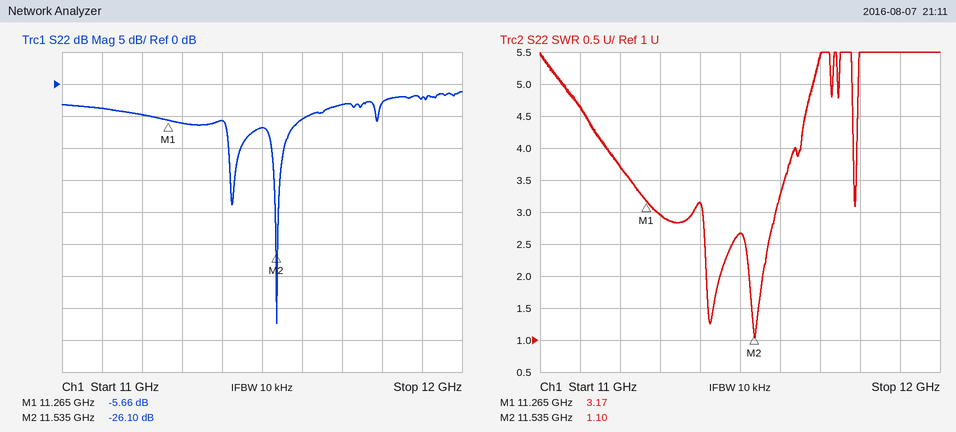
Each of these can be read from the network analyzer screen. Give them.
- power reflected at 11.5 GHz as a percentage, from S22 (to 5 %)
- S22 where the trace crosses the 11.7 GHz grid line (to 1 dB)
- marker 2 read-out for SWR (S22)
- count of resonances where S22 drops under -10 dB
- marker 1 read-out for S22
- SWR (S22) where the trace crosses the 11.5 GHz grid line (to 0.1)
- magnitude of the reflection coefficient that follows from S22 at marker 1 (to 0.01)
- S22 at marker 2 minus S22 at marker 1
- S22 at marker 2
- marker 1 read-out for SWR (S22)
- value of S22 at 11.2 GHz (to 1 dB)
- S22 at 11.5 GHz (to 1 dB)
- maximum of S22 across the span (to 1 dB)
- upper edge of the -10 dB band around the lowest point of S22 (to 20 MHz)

20 %
-3 dB
1.10
2
-5.66 dB
2.7
0.52
-20.44 dB
-26.10 dB
3.17
-5 dB
-7 dB
-1 dB
11.56 GHz
